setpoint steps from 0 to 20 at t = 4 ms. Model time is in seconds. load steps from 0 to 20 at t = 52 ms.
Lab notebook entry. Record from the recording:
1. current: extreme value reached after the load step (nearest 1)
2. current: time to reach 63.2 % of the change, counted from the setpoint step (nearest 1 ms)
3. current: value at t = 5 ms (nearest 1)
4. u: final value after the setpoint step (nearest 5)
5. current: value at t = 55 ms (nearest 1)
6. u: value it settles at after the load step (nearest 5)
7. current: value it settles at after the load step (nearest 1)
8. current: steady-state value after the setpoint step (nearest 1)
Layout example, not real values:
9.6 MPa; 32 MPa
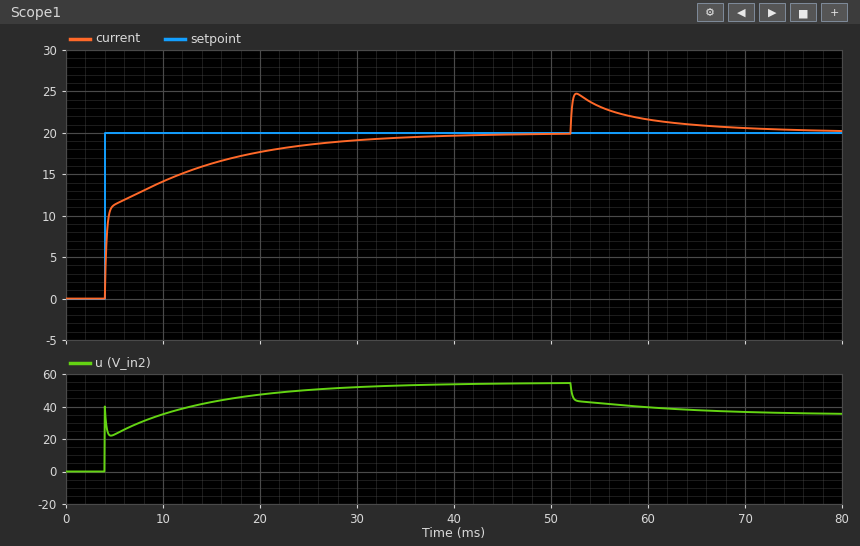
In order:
25; 3 ms; 11; 55; 23; 35; 20; 20
